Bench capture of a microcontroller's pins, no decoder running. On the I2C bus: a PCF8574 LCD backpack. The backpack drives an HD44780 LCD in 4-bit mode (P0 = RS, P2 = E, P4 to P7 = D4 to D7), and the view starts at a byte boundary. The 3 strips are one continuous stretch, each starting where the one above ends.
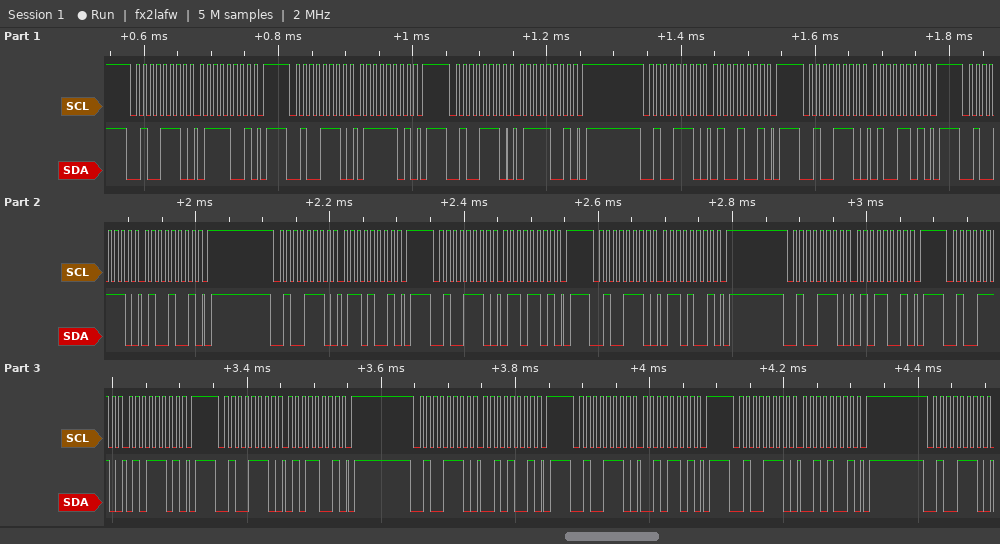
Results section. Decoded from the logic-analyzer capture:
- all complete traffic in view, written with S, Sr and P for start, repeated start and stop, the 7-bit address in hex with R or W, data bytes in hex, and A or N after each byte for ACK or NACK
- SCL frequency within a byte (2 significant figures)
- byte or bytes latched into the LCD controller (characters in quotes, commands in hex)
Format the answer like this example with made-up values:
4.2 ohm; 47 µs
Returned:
S 27W A 79 A P S 27W A 7D A P S 27W A 79 A P S 27W A 49 A P S 27W A 4D A P S 27W A 49 A P S 27W A 69 A P S 27W A 6D A P S 27W A 69 A P S 27W A 59 A P S 27W A 5D A P S 27W A 59 A P S 27W A 29 A P S 27W A 2D A P S 27W A 29 A P S 27W A; 100 kHz; 't' 'e'
